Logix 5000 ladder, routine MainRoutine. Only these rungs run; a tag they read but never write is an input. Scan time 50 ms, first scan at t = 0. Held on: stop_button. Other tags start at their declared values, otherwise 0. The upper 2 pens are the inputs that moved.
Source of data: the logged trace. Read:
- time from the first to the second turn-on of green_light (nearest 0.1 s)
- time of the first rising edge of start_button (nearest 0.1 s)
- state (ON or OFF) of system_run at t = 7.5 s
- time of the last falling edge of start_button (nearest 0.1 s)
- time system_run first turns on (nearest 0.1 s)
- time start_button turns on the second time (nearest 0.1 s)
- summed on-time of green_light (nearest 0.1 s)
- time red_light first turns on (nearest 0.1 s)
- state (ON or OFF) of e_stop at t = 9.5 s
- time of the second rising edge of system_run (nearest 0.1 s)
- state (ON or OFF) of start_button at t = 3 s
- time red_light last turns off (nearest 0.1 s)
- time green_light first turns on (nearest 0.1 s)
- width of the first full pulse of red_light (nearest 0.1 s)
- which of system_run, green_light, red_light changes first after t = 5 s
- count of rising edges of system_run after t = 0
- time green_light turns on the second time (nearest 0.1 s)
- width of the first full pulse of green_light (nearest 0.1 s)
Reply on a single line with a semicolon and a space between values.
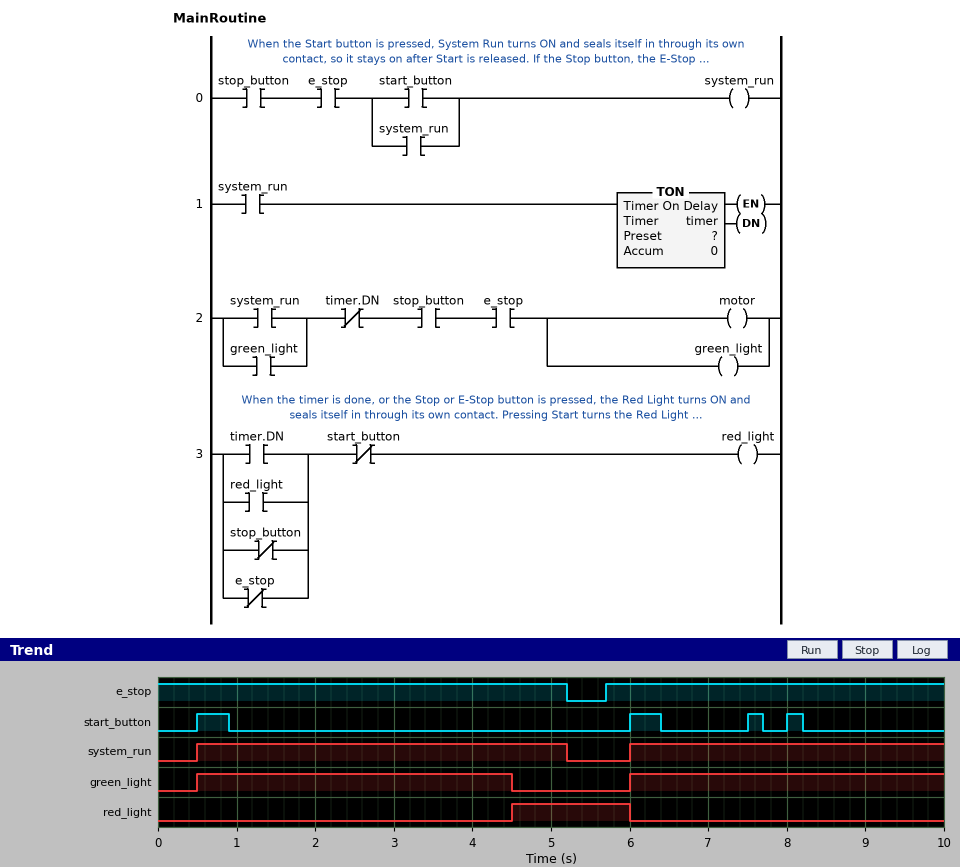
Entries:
5.5 s; 0.5 s; ON; 8.2 s; 0.5 s; 6.0 s; 8.0 s; 4.5 s; ON; 6.0 s; OFF; 6.0 s; 0.5 s; 1.5 s; system_run; 2; 6.0 s; 4.0 s
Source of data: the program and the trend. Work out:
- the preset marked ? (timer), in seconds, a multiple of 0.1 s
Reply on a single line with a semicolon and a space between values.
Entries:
4.0 s
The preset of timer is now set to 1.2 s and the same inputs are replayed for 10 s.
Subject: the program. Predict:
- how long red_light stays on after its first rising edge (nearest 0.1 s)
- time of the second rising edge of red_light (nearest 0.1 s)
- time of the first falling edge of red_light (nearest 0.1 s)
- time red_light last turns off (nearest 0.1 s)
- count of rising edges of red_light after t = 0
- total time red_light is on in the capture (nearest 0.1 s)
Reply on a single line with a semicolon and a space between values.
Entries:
4.3 s; 7.2 s; 6.0 s; 8.0 s; 4; 6.7 s
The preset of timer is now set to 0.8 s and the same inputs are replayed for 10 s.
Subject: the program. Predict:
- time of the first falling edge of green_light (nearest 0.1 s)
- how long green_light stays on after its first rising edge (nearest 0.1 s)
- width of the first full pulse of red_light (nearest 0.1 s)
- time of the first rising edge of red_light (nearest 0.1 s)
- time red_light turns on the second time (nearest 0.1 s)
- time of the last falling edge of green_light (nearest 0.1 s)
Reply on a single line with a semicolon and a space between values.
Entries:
1.3 s; 0.8 s; 4.7 s; 1.3 s; 6.8 s; 6.8 s
